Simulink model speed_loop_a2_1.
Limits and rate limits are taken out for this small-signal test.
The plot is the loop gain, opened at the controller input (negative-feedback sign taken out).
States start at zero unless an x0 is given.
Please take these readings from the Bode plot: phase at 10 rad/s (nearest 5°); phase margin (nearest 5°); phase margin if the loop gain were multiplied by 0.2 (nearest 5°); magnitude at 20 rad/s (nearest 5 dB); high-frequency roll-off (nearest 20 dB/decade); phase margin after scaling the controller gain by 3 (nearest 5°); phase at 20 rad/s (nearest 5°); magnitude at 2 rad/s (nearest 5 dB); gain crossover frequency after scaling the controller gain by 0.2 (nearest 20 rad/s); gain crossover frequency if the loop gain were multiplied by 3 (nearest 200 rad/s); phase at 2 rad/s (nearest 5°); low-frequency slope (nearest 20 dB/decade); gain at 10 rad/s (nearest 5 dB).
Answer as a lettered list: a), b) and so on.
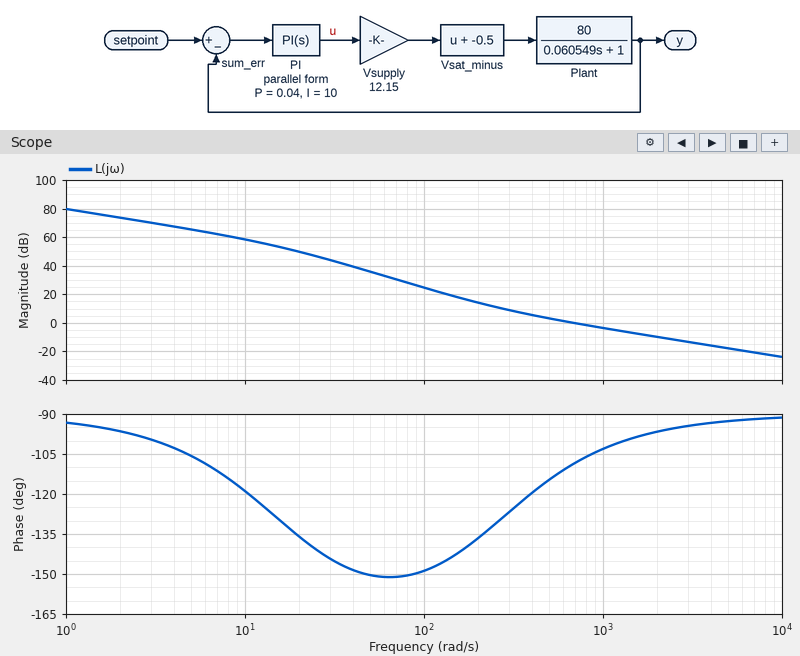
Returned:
a) -120°
b) 70°
c) 45°
d) 50 dB
e) -20 dB/decade
f) 85°
g) -135°
h) 75 dB
i) 200 rad/s
j) 2000 rad/s
k) -95°
l) -20 dB/decade
m) 60 dB
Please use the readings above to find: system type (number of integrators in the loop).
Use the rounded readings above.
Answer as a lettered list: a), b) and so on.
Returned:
a) 1
